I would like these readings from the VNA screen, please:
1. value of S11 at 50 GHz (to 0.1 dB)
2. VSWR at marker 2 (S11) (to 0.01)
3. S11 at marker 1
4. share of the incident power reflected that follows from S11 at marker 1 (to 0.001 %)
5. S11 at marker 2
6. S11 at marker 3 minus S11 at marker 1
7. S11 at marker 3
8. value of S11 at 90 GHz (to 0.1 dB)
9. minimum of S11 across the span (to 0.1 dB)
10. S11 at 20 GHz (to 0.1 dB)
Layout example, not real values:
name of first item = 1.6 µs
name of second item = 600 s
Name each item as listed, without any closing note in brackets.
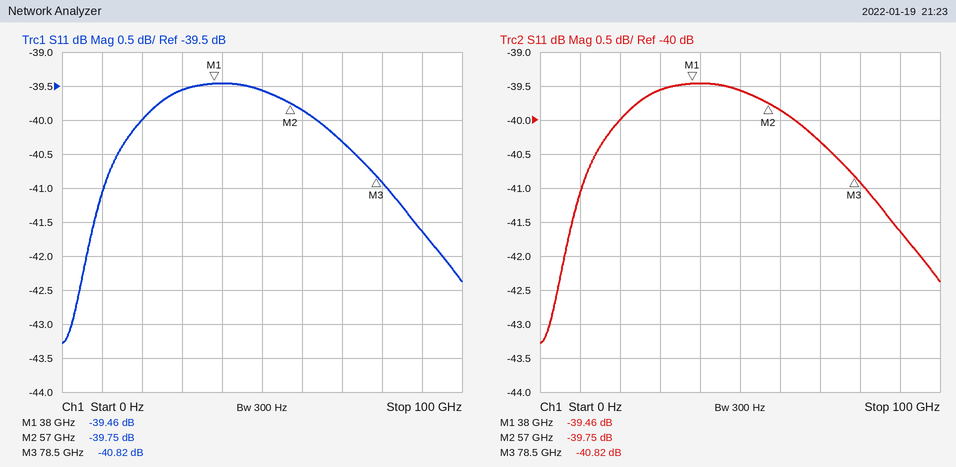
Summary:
value of S11 at 50 GHz = -39.6 dB
VSWR at marker 2 (S11) = 1.02
S11 at marker 1 = -39.46 dB
share of the incident power reflected that follows from S11 at marker 1 = 0.011 %
S11 at marker 2 = -39.75 dB
S11 at marker 3 minus S11 at marker 1 = -1.36 dB
S11 at marker 3 = -40.82 dB
value of S11 at 90 GHz = -41.6 dB
minimum of S11 across the span = -43.3 dB
S11 at 20 GHz = -40.0 dB
